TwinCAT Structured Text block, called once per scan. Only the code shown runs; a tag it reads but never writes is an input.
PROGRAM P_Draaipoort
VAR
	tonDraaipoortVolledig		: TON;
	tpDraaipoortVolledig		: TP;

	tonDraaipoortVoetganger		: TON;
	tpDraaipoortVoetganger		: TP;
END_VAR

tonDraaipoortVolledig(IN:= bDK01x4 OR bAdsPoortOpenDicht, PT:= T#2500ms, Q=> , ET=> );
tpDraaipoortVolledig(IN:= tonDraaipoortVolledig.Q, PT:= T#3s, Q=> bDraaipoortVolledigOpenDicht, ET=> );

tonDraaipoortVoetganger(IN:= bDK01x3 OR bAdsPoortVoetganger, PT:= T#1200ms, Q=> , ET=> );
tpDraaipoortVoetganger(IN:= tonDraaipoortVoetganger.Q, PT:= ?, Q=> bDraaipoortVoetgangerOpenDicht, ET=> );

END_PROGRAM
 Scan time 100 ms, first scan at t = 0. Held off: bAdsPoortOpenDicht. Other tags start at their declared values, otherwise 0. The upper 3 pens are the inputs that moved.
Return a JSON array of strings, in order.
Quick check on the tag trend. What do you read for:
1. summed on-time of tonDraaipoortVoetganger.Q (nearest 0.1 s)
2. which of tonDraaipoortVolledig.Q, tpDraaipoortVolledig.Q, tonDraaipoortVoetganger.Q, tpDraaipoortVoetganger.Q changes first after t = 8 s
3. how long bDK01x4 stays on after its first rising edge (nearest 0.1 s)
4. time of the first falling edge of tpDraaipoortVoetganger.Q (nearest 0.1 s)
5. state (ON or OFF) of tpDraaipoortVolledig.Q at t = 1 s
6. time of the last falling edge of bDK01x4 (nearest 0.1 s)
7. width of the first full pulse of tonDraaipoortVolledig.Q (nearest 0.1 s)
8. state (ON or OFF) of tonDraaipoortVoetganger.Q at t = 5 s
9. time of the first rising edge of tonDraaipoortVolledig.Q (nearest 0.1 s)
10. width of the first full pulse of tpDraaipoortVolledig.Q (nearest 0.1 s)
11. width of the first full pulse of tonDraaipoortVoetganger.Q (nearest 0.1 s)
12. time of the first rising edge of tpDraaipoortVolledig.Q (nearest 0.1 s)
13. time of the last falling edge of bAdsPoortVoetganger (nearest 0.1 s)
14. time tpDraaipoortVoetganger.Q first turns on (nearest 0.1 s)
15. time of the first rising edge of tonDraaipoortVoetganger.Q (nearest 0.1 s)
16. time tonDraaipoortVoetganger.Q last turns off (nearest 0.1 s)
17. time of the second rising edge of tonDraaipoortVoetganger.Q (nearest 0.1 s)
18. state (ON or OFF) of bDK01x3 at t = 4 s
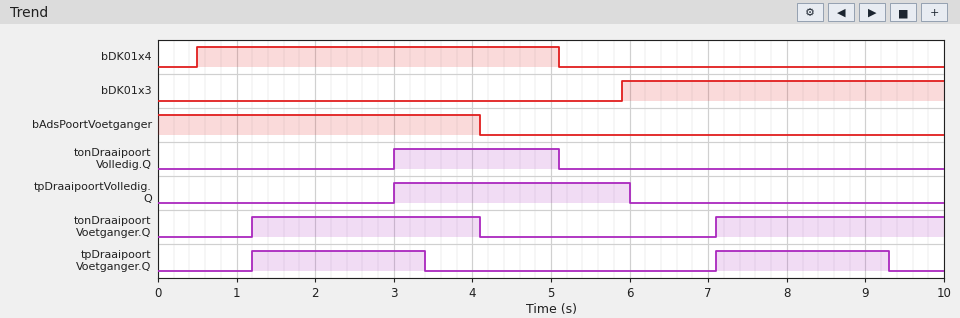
["5.8 s", "tpDraaipoortVoetganger.Q", "4.6 s", "3.4 s", "OFF", "5.1 s", "2.1 s", "OFF", "3.0 s", "3.0 s", "2.9 s", "3.0 s", "4.1 s", "1.2 s", "1.2 s", "4.1 s", "7.1 s", "OFF"]
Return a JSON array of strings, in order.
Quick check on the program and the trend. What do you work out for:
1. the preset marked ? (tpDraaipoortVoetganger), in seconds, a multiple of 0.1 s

["2.2 s"]
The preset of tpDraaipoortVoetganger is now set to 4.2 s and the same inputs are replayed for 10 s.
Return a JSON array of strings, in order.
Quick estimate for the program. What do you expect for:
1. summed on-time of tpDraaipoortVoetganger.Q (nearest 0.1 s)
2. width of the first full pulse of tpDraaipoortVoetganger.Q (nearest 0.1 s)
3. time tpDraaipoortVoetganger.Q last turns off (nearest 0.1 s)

["7.1 s", "4.2 s", "5.4 s"]
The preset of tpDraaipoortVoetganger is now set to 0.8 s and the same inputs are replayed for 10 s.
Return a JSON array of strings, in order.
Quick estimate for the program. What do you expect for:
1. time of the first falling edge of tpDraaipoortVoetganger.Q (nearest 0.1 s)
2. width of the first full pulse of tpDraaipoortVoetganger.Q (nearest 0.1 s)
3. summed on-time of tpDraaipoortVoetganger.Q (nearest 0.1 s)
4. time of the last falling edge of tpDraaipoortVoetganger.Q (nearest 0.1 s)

["2.0 s", "0.8 s", "1.6 s", "7.9 s"]
